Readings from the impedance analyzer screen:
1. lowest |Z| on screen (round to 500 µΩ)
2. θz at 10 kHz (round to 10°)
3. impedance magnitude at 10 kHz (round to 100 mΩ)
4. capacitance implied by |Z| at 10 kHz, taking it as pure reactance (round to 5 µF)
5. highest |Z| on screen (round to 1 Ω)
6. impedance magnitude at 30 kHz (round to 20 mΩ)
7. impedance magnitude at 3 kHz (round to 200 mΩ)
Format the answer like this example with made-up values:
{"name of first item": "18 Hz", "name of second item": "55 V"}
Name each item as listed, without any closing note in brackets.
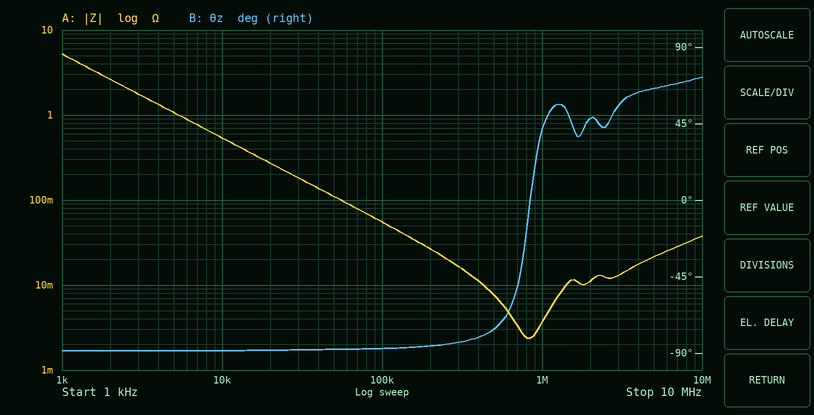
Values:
{"lowest |Z| on screen": "2.5 mΩ", "θz at 10 kHz": "-90°", "impedance magnitude at 10 kHz": "500 mΩ", "capacitance implied by |Z| at 10 kHz, taking it as pure reactance": "30 µF", "highest |Z| on screen": "5 Ω", "impedance magnitude at 30 kHz": "180 mΩ", "impedance magnitude at 3 kHz": "1.8 Ω"}
